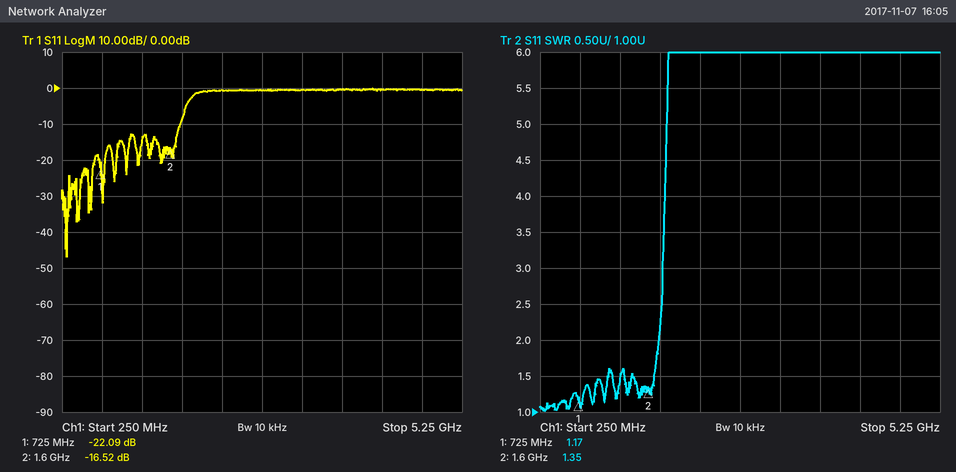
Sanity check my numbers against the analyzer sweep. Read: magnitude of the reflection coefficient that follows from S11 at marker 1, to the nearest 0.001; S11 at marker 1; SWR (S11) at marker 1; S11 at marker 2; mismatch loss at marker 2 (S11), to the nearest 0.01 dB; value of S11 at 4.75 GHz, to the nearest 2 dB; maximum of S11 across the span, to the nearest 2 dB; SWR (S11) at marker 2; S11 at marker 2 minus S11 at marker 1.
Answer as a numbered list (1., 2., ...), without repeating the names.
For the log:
1. 0.079
2. -22.09 dB
3. 1.17
4. -16.52 dB
5. 0.10 dB
6. 0 dB
7. 0 dB
8. 1.35
9. 5.57 dB
